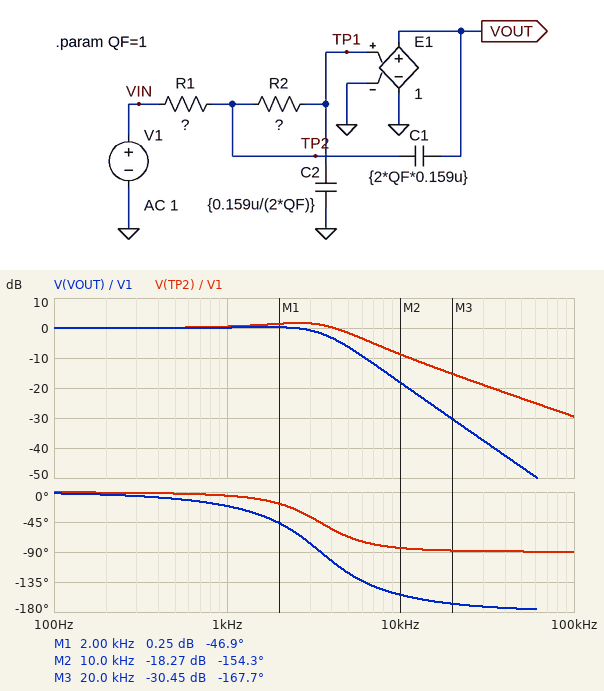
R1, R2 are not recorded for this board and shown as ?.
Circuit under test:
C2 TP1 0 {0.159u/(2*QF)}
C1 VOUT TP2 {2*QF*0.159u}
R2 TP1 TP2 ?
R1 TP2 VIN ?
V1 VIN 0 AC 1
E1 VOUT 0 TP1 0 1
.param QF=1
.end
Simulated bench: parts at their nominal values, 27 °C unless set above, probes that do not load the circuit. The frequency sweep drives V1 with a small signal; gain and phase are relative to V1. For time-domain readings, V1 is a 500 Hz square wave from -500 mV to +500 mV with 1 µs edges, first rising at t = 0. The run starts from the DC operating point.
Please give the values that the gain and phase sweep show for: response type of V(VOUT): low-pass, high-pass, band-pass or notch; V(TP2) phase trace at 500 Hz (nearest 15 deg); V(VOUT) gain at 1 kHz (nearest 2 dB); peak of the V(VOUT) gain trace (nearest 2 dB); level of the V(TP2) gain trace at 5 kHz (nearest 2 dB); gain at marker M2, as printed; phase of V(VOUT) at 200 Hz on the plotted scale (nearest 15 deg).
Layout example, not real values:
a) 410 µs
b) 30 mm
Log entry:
a) low-pass
b) 0 deg
c) 0 dB
d) 0 dB
e) -2 dB
f) -18.27 dB
g) 0 deg
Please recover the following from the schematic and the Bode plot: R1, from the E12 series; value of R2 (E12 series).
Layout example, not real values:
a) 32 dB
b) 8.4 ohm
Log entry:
a) 150 Ω
b) 560 Ω
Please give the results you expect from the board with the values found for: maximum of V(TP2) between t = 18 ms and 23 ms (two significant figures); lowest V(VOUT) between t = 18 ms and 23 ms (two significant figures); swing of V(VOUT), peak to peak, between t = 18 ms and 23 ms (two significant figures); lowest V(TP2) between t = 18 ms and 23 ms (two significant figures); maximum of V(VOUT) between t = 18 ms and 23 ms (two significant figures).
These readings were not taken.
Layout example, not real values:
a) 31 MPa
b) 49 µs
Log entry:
a) 680 mV
b) -590 mV
c) 1.2 V
d) -680 mV
e) 590 mV
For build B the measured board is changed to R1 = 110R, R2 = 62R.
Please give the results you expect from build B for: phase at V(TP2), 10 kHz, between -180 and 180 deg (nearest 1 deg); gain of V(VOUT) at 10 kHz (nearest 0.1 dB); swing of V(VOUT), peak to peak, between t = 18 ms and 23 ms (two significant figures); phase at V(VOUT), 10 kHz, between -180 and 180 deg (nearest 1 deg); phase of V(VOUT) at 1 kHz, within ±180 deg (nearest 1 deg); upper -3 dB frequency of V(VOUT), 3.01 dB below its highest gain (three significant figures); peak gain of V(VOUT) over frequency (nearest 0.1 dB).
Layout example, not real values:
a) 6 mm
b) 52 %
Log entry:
a) -52 deg
b) 0.8 dB
c) 1.3 V
d) -70 deg
e) -5 deg
f) 14.1 kHz
g) 1.0 dB
